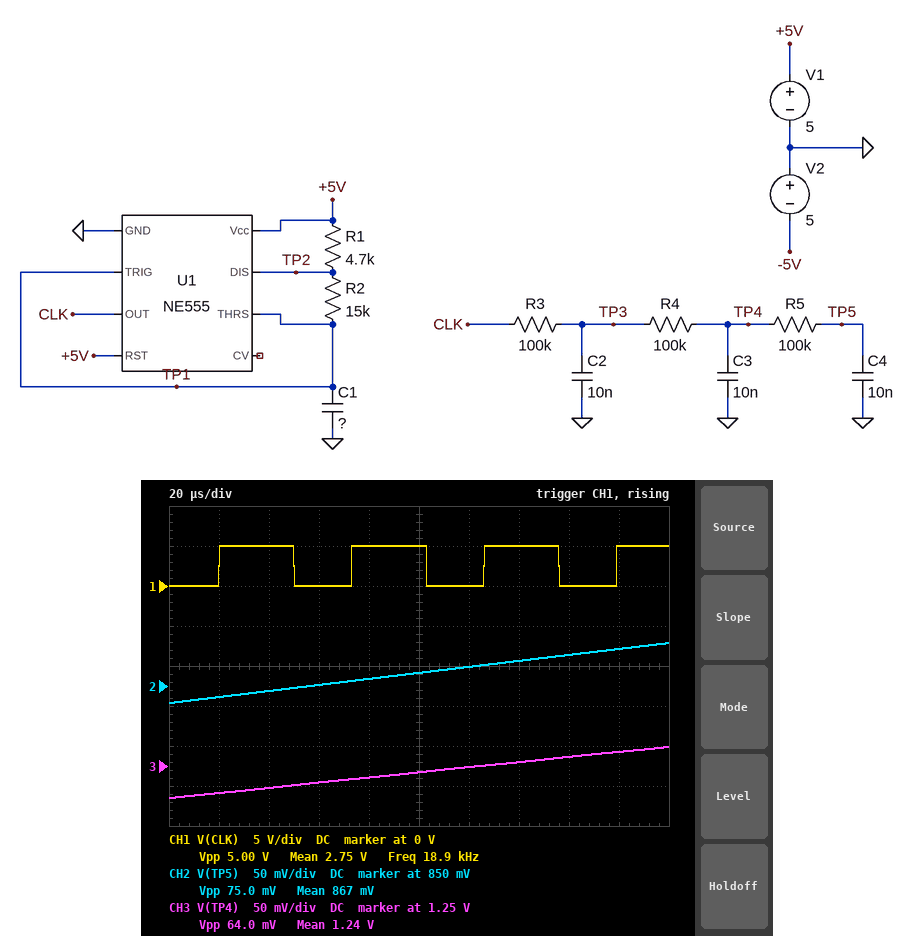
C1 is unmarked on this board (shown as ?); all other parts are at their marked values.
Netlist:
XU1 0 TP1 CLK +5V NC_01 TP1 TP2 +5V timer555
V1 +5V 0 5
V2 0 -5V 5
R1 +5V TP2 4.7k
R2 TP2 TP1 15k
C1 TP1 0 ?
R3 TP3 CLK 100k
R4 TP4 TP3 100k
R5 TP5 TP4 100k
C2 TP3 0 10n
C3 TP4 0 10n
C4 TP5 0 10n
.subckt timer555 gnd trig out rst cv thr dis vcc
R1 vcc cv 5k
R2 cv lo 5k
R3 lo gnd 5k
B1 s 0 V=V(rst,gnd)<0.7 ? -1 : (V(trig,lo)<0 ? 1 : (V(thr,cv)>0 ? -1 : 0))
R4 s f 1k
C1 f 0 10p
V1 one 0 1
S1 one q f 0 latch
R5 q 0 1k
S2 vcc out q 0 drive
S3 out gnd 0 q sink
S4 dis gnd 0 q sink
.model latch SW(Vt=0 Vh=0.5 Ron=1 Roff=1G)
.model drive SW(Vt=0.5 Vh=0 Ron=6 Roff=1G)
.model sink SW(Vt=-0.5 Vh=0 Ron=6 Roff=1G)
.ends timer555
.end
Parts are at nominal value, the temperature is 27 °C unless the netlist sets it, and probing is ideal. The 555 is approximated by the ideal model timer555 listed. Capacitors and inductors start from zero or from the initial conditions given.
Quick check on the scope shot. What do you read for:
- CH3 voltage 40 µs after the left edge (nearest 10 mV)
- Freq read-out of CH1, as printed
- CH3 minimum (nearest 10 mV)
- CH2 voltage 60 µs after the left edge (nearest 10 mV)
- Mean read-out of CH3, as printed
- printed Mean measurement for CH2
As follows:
1.22 V
18.9 kHz
1.21 V
850 mV
1.24 V
867 mV
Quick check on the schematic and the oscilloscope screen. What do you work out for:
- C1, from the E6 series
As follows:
2.2 nF
